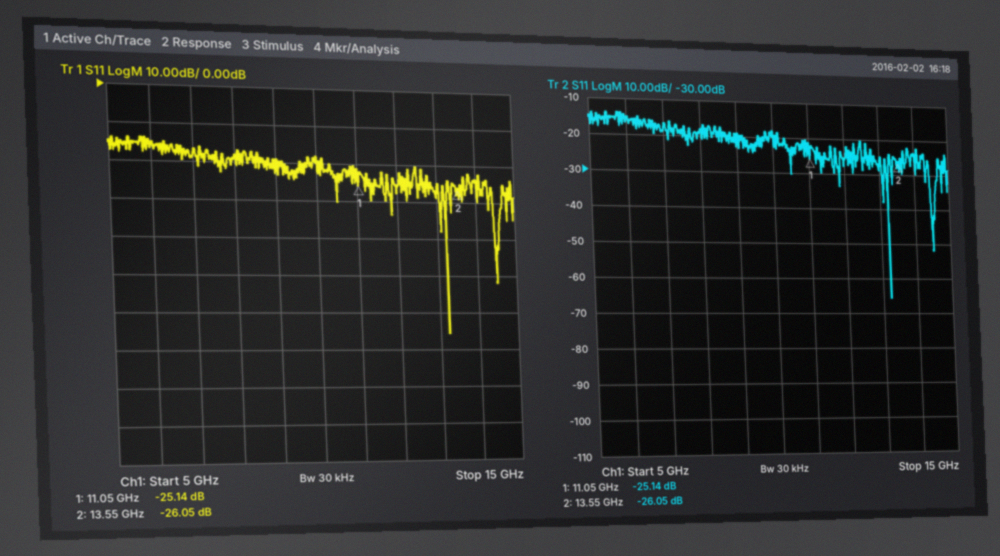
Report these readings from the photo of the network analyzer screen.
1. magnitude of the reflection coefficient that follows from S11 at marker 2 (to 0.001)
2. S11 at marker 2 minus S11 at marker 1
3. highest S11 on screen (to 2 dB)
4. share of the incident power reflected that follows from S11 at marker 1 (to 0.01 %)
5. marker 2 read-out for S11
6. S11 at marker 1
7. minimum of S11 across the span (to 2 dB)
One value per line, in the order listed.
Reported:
0.050
-0.91 dB
-14 dB
0.31 %
-26.05 dB
-25.14 dB
-66 dB
